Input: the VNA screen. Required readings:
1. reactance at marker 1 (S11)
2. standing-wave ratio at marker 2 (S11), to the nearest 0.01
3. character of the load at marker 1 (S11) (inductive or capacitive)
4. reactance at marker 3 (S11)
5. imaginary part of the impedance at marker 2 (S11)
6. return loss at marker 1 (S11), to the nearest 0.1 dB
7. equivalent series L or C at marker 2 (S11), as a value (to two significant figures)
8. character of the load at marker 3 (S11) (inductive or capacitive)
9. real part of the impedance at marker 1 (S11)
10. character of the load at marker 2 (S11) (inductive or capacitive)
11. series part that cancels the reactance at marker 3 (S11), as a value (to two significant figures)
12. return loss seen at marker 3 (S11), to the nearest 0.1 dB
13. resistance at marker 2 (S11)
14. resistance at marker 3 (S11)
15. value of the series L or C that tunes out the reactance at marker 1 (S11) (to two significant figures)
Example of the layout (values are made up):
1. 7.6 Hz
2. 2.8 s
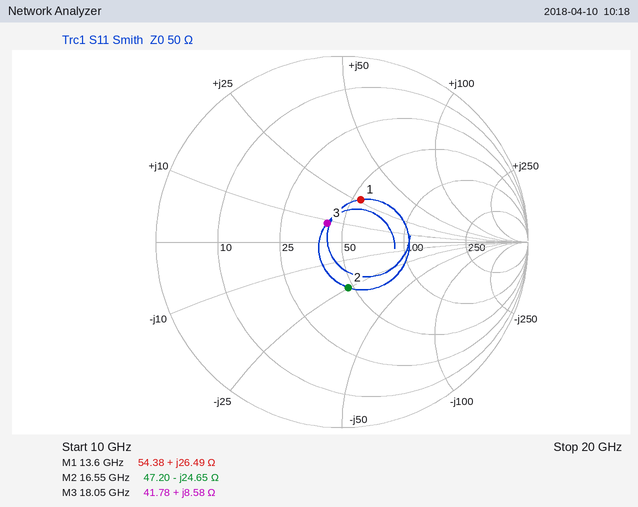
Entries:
1. +26.49 Ω
2. 1.66
3. inductive
4. +8.58 Ω
5. -24.65 Ω
6. 12.1 dB
7. 390 fF
8. inductive
9. 54.38 Ω
10. capacitive
11. 1.0 pF
12. 17.8 dB
13. 47.20 Ω
14. 41.78 Ω
15. 440 fF
